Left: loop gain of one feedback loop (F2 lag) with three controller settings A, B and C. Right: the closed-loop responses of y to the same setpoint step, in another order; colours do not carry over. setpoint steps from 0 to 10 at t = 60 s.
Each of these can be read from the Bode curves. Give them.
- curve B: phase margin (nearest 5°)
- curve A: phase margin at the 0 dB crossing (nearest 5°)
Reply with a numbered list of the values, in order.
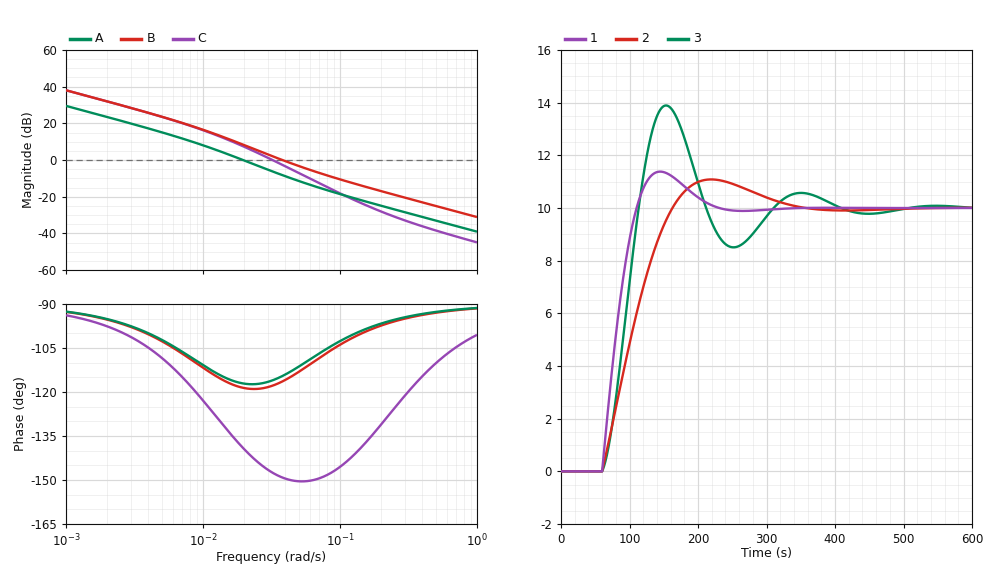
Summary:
1. 65°
2. 65°
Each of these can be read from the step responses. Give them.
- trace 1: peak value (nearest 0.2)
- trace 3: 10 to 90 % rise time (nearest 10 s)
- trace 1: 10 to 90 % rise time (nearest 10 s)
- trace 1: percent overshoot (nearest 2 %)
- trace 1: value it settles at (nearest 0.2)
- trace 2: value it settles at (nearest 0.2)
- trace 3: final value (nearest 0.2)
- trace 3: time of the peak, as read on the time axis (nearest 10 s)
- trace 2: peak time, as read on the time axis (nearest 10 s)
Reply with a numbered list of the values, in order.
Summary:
1. 11.4
2. 40 s
3. 40 s
4. 14 %
5. 10.0
6. 10.0
7. 10.0
8. 150 s
9. 220 s
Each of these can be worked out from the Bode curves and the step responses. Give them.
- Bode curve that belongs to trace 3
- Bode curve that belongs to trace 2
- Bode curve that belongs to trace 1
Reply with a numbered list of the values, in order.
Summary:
1. C
2. A
3. B
